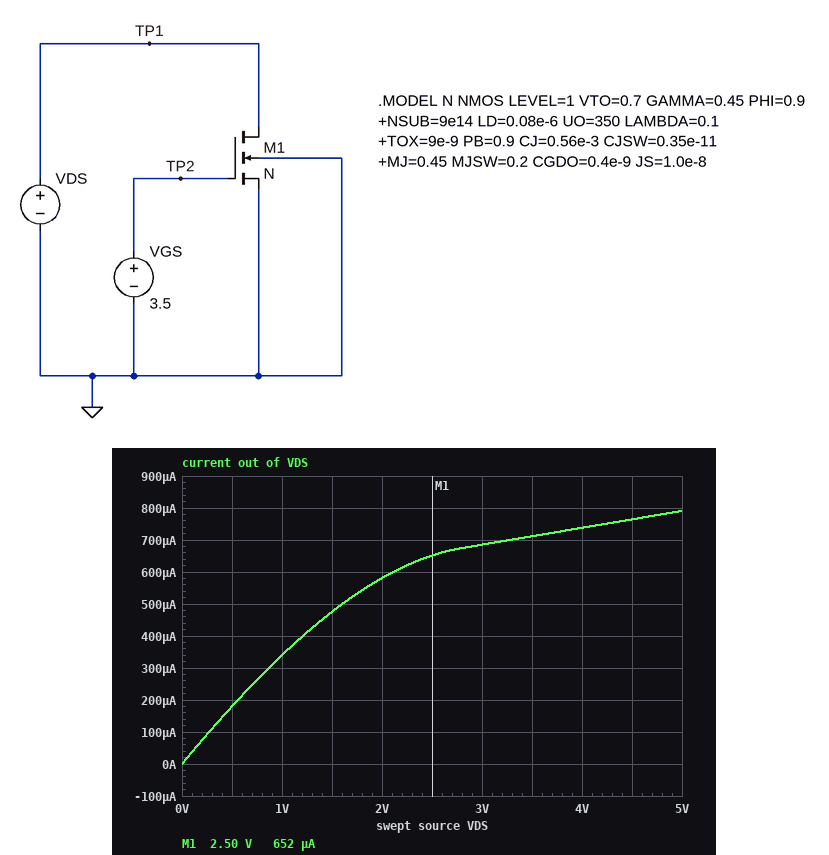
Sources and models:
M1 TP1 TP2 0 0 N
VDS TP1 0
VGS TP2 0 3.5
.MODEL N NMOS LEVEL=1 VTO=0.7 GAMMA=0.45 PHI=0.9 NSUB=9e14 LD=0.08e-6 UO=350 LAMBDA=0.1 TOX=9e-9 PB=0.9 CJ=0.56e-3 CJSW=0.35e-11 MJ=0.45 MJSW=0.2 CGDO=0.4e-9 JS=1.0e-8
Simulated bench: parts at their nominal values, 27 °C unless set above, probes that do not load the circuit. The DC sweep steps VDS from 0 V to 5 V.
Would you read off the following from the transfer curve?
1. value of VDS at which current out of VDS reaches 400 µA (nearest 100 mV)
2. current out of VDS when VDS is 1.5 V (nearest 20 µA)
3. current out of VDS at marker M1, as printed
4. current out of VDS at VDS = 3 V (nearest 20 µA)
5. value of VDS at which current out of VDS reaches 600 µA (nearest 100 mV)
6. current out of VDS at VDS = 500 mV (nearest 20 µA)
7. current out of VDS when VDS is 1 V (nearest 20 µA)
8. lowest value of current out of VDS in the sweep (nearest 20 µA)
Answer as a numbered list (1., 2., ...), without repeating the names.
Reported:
1. 1.2 V
2. 480 µA
3. 652 µA
4. 680 µA
5. 2.1 V
6. 180 µA
7. 340 µA
8. 0 A
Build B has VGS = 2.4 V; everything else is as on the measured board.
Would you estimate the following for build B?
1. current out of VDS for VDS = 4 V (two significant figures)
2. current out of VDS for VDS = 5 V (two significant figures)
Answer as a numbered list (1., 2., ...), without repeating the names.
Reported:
1. 270 µA
2. 290 µA
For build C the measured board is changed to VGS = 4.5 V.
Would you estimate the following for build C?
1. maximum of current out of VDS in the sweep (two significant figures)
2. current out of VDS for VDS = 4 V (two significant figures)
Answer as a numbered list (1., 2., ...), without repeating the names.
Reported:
1. 1.5 mA
2. 1.4 mA
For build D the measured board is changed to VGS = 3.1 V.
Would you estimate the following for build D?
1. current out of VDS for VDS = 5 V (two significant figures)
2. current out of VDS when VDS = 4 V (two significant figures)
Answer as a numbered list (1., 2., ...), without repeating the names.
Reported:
1. 580 µA
2. 540 µA
